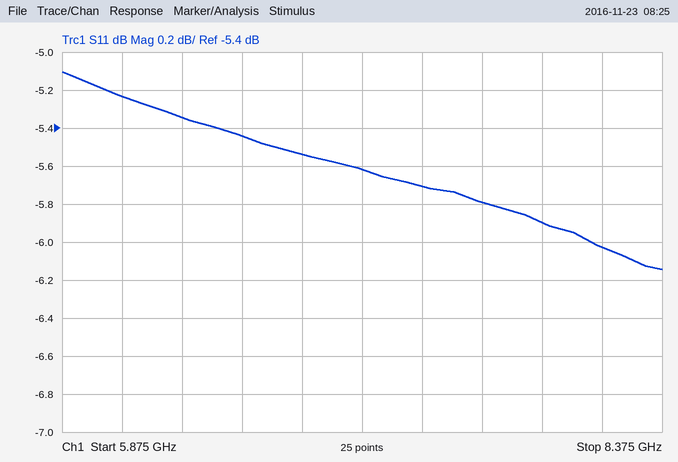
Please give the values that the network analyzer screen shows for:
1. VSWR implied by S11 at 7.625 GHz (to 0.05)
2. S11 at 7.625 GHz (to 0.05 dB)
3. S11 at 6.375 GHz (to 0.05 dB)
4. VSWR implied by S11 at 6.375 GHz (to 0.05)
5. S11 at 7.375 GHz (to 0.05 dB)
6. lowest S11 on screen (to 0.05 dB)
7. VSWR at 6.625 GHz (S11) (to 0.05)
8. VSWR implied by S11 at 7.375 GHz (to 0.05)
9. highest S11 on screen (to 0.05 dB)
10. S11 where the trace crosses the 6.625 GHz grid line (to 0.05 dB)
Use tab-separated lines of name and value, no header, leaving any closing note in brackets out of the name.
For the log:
VSWR implied by S11 at 7.625 GHz	3.10
S11 at 7.625 GHz	-5.80 dB
S11 at 6.375 GHz	-5.35 dB
VSWR implied by S11 at 6.375 GHz	3.35
S11 at 7.375 GHz	-5.70 dB
lowest S11 on screen	-6.15 dB
VSWR at 6.625 GHz (S11)	3.30
VSWR implied by S11 at 7.375 GHz	3.15
highest S11 on screen	-5.10 dB
S11 where the trace crosses the 6.625 GHz grid line	-5.45 dB
